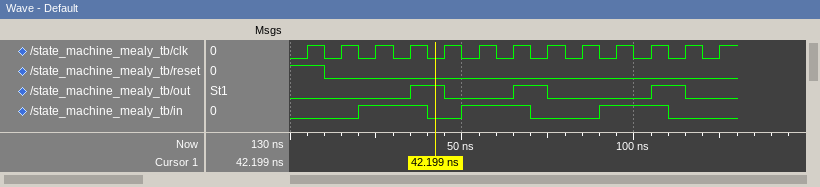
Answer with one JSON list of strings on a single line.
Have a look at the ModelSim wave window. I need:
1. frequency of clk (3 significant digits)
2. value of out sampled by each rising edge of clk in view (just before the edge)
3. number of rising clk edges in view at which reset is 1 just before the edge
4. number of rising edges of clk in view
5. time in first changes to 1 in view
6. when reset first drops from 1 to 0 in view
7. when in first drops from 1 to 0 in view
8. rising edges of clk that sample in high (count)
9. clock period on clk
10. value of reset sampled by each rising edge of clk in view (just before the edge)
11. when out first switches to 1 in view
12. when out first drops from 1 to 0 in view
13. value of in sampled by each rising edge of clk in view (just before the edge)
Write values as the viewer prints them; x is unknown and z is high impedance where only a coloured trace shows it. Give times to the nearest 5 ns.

["100 MHz", "0 0 0 0 1 0 0 1 0 0 0 1 0", "1", "13", "20 ns", "10 ns", "40 ns", "6", "10 ns", "1 0 0 0 0 0 0 0 0 0 0 0 0", "35 ns", "45 ns", "0 0 1 1 0 1 1 0 0 1 1 0 0"]
